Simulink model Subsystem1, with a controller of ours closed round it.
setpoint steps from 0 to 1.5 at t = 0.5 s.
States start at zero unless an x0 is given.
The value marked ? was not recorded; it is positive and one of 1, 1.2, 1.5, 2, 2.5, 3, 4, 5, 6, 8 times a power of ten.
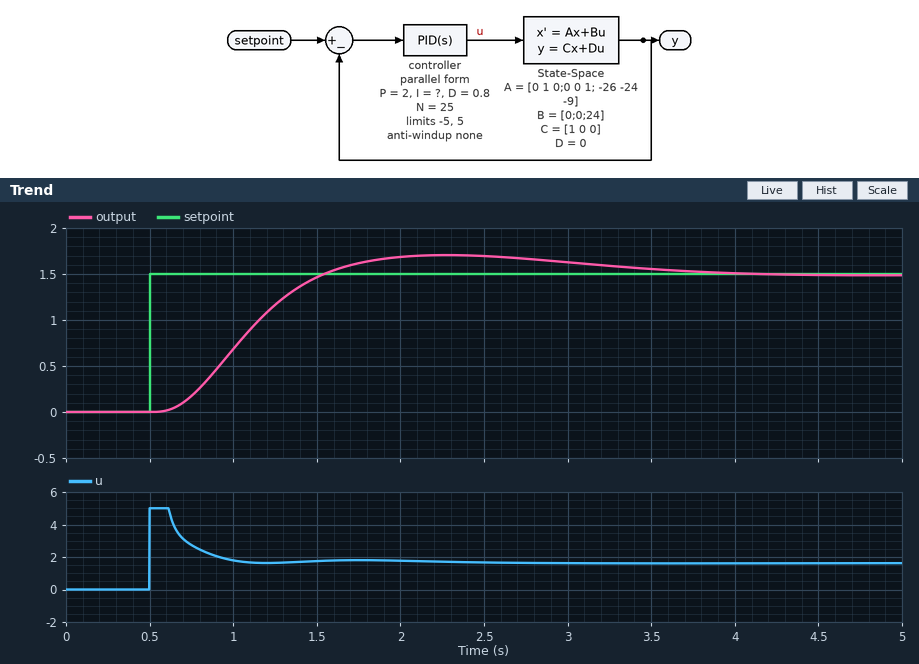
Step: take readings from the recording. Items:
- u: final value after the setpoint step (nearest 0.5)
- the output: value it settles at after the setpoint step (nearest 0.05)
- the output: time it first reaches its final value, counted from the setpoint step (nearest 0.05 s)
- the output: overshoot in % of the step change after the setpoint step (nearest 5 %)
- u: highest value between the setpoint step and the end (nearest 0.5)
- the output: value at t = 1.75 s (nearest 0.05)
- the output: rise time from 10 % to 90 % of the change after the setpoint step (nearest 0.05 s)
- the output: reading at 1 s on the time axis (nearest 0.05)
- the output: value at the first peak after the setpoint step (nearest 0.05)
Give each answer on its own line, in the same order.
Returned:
1.5
1.50
1.05 s
15 %
5.0
1.60
0.65 s
0.70
1.70
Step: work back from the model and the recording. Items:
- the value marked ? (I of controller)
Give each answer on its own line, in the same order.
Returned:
3
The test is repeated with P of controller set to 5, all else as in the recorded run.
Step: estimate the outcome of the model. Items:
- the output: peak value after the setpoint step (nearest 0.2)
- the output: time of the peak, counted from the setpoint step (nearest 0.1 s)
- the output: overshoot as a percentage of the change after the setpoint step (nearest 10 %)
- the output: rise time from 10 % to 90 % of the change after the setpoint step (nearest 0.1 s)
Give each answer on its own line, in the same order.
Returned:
1.8
1.0 s
20 %
0.4 s
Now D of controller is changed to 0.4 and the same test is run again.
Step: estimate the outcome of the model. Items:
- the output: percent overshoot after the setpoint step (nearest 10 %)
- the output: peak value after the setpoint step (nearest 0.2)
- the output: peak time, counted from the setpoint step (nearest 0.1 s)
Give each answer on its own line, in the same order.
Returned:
20 %
1.8
1.3 s
